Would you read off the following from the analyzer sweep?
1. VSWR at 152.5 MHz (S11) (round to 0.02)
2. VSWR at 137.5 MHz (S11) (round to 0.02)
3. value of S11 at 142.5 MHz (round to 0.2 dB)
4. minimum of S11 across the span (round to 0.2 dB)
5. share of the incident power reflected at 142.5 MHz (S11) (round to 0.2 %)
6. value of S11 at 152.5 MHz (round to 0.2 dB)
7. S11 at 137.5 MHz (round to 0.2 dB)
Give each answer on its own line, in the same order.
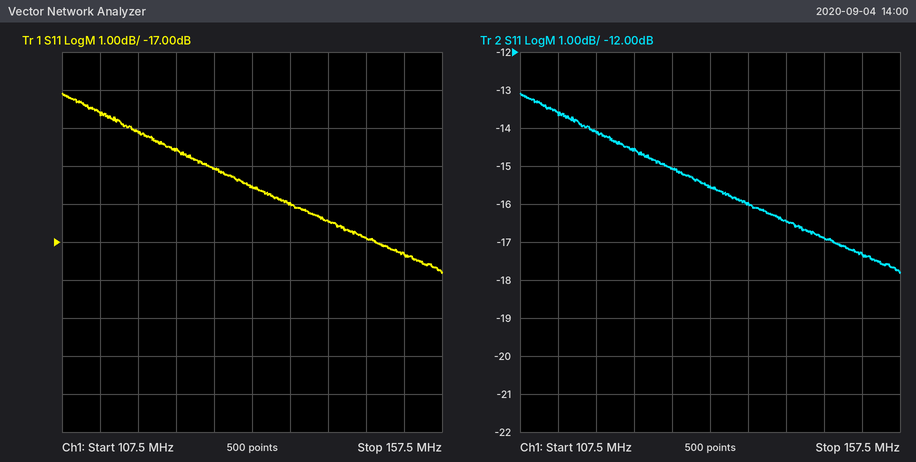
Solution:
1.32
1.38
-16.4 dB
-17.8 dB
2.2 %
-17.4 dB
-16.0 dB
